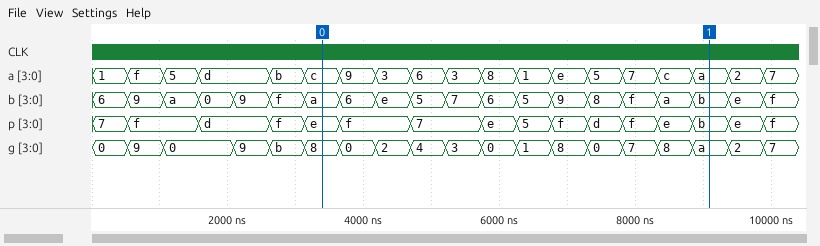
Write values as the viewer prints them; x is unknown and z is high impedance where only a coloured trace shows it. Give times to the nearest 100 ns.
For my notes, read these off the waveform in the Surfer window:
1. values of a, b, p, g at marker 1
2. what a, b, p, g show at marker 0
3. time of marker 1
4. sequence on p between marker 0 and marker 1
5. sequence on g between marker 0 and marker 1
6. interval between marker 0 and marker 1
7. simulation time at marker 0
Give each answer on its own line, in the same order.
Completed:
a=a, b=b, p=b, g=a
a=c, b=a, p=e, g=8
9100 ns
e, f, 7, e, 5, f, d, f, e, b
8, 0, 2, 4, 3, 0, 1, 8, 0, 7, 8, a
5700 ns
3400 ns
